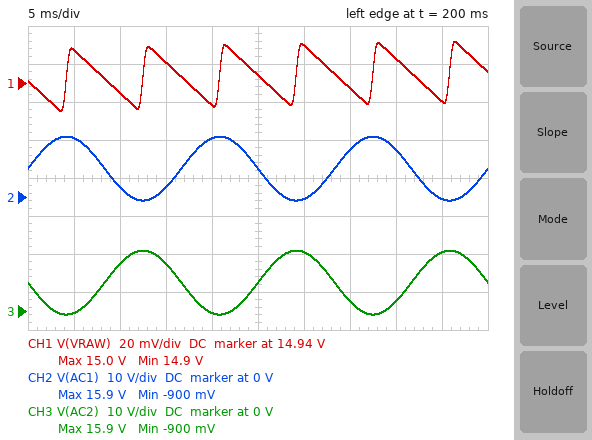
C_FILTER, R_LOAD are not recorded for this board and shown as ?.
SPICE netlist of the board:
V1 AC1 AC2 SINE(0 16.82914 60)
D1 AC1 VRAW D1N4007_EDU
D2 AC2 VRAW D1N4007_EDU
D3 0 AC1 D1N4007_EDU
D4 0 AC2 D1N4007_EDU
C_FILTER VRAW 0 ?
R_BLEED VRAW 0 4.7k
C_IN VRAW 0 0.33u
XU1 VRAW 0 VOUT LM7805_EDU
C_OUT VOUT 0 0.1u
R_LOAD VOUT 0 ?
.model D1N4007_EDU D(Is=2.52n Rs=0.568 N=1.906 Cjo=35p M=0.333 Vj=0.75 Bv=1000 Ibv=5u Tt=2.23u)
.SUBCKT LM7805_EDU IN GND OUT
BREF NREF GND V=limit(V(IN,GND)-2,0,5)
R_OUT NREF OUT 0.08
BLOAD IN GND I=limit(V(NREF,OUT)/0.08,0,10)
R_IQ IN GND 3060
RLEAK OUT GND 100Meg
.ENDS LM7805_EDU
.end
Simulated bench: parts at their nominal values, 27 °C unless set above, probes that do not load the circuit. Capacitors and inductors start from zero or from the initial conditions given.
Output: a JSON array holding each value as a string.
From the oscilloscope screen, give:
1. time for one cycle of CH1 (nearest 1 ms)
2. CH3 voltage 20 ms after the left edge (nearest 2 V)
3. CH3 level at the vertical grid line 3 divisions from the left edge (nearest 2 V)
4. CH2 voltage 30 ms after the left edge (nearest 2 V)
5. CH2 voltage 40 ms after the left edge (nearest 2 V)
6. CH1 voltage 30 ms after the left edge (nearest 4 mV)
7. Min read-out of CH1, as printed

["8 ms", "0 V", "12 V", "0 V", "12 V", "14.960 V", "14.9 V"]
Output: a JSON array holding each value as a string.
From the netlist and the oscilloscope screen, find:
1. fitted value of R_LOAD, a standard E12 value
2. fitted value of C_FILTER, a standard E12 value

["2.7 kΩ", "2.2 mF"]
